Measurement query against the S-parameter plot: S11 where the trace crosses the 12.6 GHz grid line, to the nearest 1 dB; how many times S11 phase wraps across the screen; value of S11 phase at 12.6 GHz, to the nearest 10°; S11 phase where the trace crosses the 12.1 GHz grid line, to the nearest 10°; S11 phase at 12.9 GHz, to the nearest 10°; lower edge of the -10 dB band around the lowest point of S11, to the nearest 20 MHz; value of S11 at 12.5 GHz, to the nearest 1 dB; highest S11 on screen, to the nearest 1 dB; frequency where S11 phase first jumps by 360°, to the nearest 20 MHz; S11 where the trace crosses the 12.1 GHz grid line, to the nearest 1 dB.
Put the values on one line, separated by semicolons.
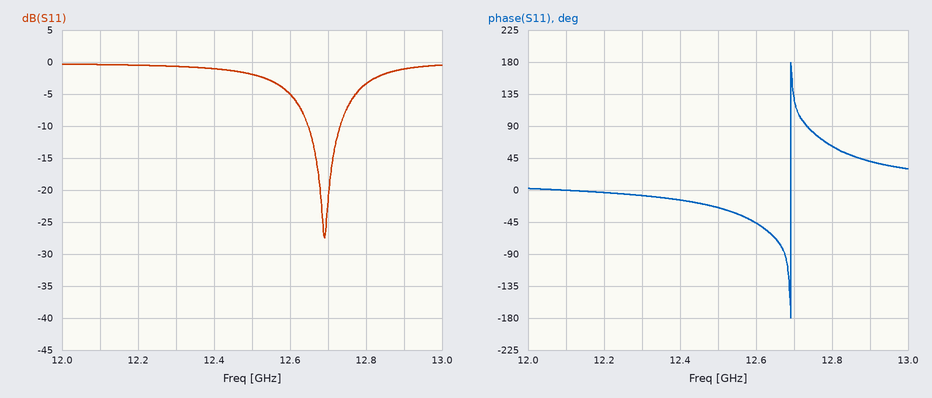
-5 dB; 1; -50°; 0°; 40°; 12.64 GHz; -2 dB; 0 dB; 12.70 GHz; 0 dB
